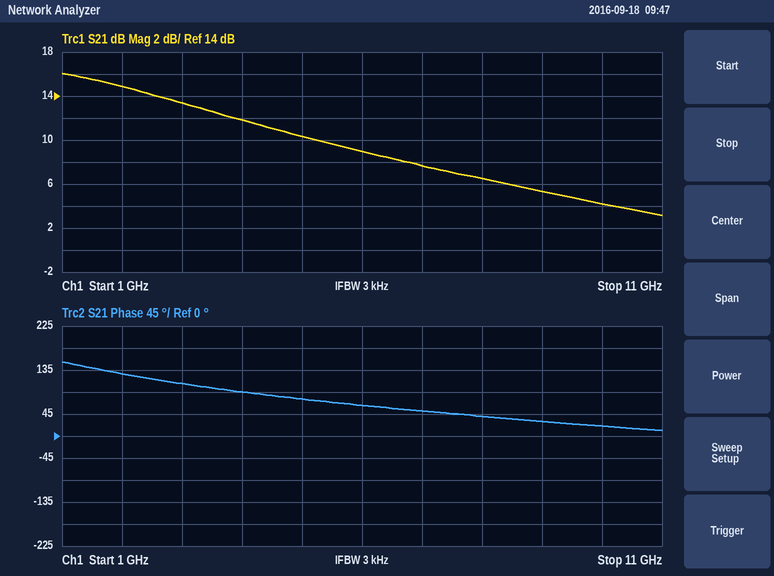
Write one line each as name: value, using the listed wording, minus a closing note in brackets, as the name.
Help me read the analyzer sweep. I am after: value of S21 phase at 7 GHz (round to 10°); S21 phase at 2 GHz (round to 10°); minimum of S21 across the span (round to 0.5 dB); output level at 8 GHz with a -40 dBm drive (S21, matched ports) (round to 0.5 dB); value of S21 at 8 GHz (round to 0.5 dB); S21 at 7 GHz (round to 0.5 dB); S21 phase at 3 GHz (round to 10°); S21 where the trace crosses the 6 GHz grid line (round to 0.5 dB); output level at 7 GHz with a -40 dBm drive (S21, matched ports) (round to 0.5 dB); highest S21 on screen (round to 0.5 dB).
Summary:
value of S21 phase at 7 GHz: 50°
S21 phase at 2 GHz: 130°
minimum of S21 across the span: 3.0 dB
output level at 8 GHz with a -40 dBm drive (S21, matched ports): -33.5 dBm
value of S21 at 8 GHz: 6.5 dB
S21 at 7 GHz: 7.5 dB
S21 phase at 3 GHz: 110°
S21 where the trace crosses the 6 GHz grid line: 9.0 dB
output level at 7 GHz with a -40 dBm drive (S21, matched ports): -32.5 dBm
highest S21 on screen: 16.0 dB
